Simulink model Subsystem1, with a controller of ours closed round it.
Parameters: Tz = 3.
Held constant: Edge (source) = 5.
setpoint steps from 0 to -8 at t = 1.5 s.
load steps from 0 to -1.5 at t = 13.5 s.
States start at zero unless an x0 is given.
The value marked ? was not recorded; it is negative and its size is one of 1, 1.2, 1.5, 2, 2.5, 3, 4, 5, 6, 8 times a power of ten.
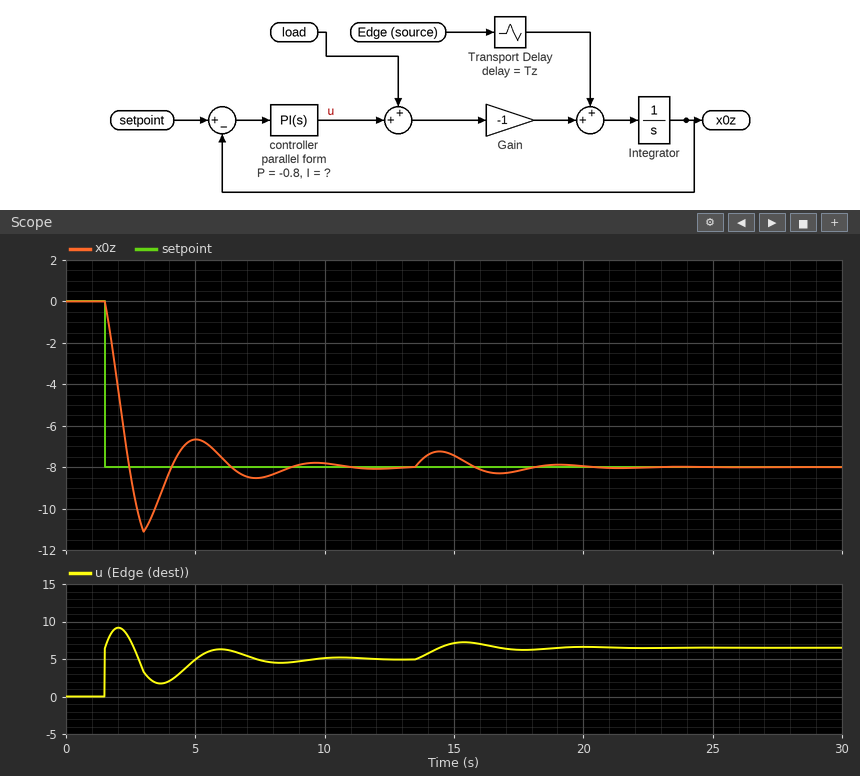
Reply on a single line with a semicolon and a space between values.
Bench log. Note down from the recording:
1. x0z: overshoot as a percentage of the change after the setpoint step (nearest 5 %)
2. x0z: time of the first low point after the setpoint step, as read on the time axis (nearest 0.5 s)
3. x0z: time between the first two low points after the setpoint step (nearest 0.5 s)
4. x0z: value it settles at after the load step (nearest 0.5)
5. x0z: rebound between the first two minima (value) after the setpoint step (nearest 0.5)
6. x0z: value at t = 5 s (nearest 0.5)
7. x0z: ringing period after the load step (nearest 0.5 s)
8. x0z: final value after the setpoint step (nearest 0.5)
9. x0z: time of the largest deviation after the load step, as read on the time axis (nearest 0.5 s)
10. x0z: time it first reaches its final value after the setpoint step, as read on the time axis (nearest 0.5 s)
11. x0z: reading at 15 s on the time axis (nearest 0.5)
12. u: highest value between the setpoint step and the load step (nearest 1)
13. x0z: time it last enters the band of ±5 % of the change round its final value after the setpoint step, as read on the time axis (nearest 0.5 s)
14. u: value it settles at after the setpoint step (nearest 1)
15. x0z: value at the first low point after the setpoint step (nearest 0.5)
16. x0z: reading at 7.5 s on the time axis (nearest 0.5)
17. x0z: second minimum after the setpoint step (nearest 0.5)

40 %; 3.0 s; 4.5 s; -8.0; -6.5; -6.5; 4.5 s; -8.0; 14.5 s; 2.5 s; -7.5; 9; 8.0 s; 5; -11.0; -8.5; -8.5
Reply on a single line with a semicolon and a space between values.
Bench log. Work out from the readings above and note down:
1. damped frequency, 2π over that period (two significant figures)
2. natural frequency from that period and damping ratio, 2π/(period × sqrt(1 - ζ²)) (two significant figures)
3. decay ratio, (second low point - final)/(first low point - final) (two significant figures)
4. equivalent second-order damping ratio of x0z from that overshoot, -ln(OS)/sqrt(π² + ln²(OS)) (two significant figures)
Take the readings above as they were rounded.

1.4 rad/s; 1.5 rad/s; 0.17; 0.28
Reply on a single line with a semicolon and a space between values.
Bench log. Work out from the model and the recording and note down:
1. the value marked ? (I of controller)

-2
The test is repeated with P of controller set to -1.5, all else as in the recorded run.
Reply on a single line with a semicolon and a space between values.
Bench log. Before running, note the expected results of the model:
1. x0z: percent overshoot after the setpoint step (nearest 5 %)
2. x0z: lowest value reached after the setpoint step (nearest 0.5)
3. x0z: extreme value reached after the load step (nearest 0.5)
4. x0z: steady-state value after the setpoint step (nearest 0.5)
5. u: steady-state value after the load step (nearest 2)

25 %; -10.0; -7.5; -8.0; 6
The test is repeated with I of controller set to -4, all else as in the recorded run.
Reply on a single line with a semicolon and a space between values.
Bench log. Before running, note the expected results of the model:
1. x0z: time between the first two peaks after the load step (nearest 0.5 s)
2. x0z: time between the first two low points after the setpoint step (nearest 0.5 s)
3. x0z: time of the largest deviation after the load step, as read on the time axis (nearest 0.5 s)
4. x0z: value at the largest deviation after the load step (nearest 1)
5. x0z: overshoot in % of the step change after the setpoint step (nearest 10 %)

3.0 s; 3.0 s; 14.0 s; -7; 60 %
